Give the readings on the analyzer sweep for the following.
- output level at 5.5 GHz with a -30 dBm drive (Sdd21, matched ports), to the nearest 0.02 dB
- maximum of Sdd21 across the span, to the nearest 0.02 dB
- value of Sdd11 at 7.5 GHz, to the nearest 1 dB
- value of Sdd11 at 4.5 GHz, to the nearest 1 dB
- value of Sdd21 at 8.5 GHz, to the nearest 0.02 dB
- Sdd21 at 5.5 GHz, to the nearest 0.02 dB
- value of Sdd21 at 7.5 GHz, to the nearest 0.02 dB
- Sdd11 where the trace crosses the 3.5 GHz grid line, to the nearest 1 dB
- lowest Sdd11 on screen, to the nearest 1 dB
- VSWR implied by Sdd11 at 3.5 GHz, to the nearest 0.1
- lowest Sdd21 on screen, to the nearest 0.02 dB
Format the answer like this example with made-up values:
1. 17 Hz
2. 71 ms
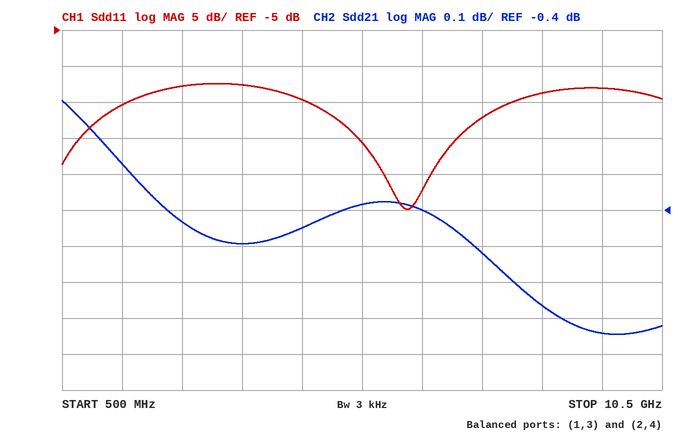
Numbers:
1. -30.38 dBm
2. -0.10 dB
3. -17 dB
4. -15 dB
5. -0.66 dB
6. -0.38 dB
7. -0.52 dB
8. -13 dB
9. -30 dB
10. 1.6
11. -0.74 dB
